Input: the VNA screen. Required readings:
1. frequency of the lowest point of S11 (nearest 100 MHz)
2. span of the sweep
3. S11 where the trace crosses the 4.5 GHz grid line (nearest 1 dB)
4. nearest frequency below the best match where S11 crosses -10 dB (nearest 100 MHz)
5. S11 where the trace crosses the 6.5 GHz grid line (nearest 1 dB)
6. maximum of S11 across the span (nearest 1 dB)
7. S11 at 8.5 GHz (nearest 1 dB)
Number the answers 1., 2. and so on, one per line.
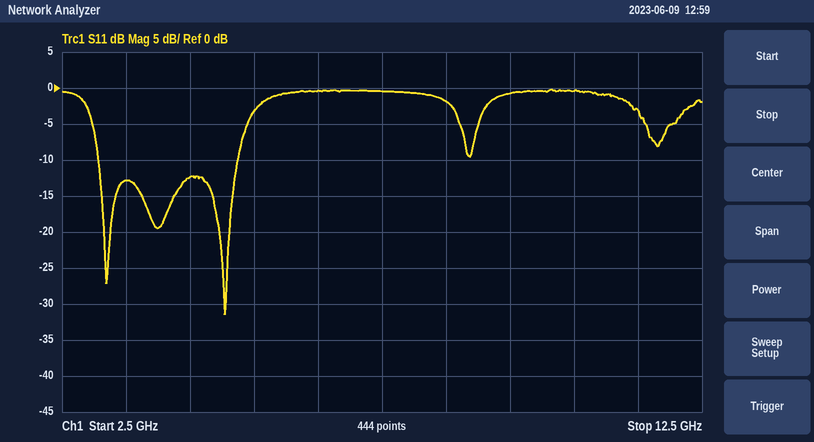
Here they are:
1. 5.0 GHz
2. 10 GHz
3. -12 dB
4. 3.1 GHz
5. 0 dB
6. 0 dB
7. -2 dB
